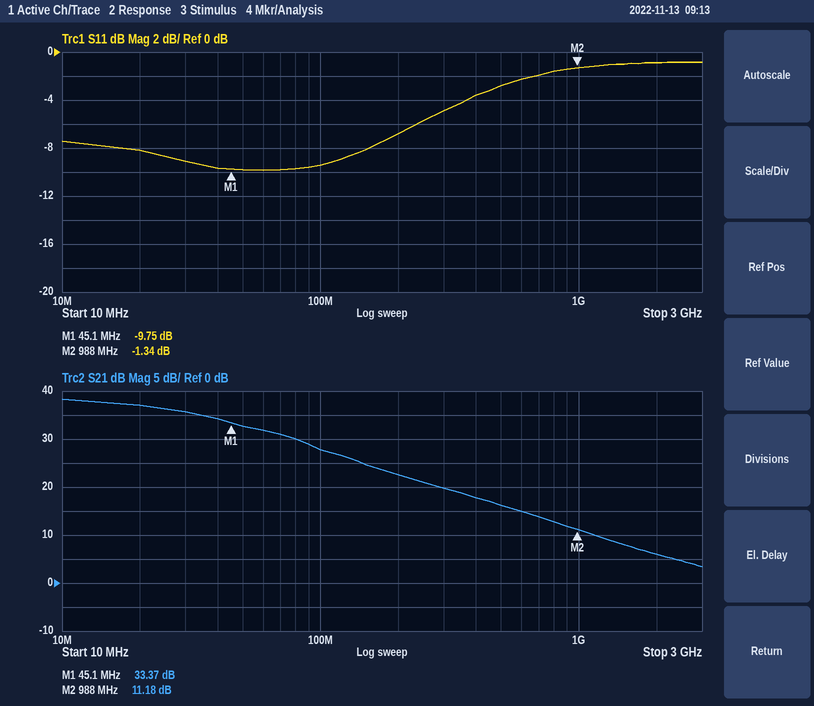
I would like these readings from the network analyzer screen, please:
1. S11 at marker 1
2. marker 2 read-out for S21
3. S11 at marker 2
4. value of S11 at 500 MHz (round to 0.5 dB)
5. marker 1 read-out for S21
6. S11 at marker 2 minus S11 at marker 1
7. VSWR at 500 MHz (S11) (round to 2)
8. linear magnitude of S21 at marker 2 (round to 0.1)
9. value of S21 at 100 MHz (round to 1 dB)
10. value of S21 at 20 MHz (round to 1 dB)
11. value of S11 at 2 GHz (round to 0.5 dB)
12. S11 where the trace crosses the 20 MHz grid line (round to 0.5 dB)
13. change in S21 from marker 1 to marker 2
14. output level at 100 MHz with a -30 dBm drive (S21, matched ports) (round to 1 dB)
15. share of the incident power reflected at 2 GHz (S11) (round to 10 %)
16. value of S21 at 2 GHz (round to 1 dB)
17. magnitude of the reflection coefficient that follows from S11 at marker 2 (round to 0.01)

-9.75 dB
11.18 dB
-1.34 dB
-3.0 dB
33.37 dB
8.41 dB
6
3.6
28 dB
37 dB
-1.0 dB
-8.0 dB
-22.19 dB
-2 dBm
80 %
6 dB
0.86
